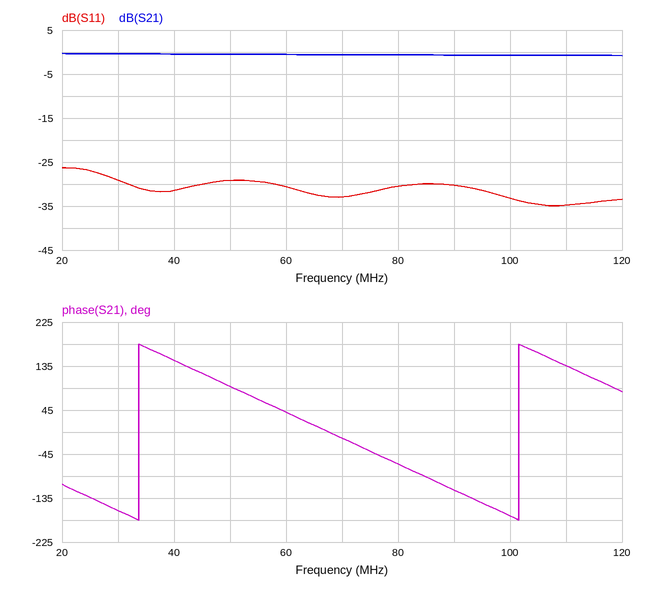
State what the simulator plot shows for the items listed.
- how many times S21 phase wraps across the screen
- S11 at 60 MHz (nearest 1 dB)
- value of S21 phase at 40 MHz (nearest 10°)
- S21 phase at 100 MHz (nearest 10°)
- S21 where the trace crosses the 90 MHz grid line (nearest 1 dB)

2
-31 dB
150°
-170°
-1 dB
